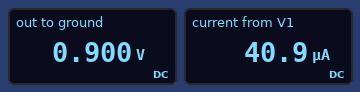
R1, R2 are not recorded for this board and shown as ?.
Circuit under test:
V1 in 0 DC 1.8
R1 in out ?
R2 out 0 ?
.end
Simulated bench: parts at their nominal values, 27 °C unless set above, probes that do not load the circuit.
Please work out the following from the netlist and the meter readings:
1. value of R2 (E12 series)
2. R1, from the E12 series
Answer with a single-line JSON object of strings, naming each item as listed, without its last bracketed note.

{"value of R2": "22 kΩ", "R1, from the E12 series": "22 kΩ"}
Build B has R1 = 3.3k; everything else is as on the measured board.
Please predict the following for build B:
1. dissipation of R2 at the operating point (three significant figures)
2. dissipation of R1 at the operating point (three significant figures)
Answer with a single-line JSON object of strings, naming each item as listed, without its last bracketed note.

{"dissipation of R2 at the operating point": "111 µW", "dissipation of R1 at the operating point": "16.7 µW"}
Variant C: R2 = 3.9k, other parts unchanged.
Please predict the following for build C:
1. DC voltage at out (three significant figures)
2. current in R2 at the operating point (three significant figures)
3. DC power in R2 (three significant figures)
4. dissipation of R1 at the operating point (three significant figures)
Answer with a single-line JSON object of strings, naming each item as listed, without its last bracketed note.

{"DC voltage at out": "271 mV", "current in R2 at the operating point": "69.5 µA", "DC power in R2": "18.8 µW", "dissipation of R1 at the operating point": "106 µW"}
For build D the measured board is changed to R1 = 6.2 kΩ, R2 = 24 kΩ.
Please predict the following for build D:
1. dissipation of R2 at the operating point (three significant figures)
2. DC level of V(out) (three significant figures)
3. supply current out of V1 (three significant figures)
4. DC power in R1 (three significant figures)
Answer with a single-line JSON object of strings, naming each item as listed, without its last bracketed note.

{"dissipation of R2 at the operating point": "85.3 µW", "DC level of V(out)": "1.43 V", "supply current out of V1": "59.6 µA", "DC power in R1": "22.0 µW"}
